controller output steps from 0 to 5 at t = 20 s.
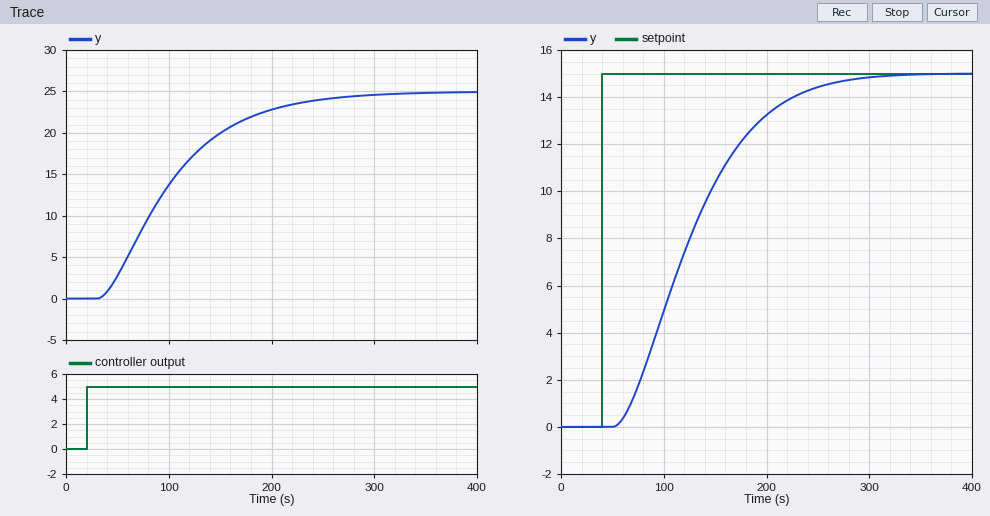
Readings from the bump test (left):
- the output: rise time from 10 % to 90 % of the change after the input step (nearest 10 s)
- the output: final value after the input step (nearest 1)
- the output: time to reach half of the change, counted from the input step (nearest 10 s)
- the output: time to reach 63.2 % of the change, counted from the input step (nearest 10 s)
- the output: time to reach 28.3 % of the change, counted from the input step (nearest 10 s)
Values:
140 s
25
70 s
90 s
50 s
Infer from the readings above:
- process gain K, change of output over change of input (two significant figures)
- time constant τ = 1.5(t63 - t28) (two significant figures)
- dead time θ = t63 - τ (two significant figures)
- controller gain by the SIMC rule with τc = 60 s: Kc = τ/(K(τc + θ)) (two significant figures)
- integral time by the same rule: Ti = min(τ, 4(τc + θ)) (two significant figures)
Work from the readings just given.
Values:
5.0
60 s
30 s
0.13
60 s
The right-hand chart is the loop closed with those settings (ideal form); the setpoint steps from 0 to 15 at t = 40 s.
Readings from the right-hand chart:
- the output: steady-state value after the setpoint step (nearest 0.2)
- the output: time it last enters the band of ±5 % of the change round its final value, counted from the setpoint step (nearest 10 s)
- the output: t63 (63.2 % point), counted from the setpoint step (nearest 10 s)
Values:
15.0
200 s
100 s
